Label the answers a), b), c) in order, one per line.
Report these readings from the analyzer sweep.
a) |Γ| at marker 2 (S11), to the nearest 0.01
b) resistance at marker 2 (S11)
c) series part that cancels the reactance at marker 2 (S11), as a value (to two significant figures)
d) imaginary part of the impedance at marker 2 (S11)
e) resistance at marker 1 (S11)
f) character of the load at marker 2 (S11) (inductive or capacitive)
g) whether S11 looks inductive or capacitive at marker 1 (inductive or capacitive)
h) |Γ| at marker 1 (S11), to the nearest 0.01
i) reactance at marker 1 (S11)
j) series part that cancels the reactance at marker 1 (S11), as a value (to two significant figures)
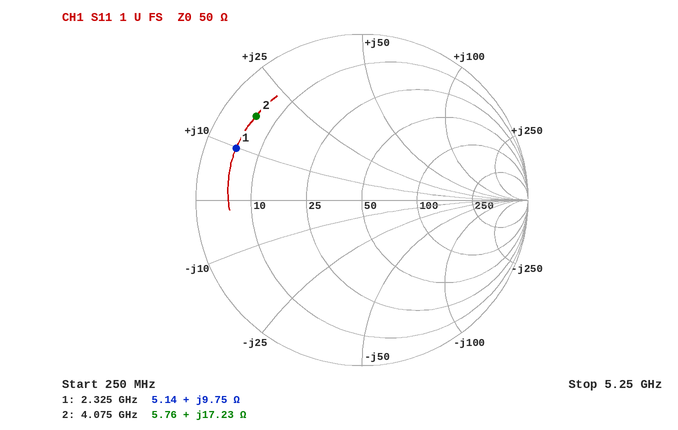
a) 0.81
b) 5.76 Ω
c) 2.3 pF
d) +17.23 Ω
e) 5.14 Ω
f) inductive
g) inductive
h) 0.82
i) +9.75 Ω
j) 7.0 pF
